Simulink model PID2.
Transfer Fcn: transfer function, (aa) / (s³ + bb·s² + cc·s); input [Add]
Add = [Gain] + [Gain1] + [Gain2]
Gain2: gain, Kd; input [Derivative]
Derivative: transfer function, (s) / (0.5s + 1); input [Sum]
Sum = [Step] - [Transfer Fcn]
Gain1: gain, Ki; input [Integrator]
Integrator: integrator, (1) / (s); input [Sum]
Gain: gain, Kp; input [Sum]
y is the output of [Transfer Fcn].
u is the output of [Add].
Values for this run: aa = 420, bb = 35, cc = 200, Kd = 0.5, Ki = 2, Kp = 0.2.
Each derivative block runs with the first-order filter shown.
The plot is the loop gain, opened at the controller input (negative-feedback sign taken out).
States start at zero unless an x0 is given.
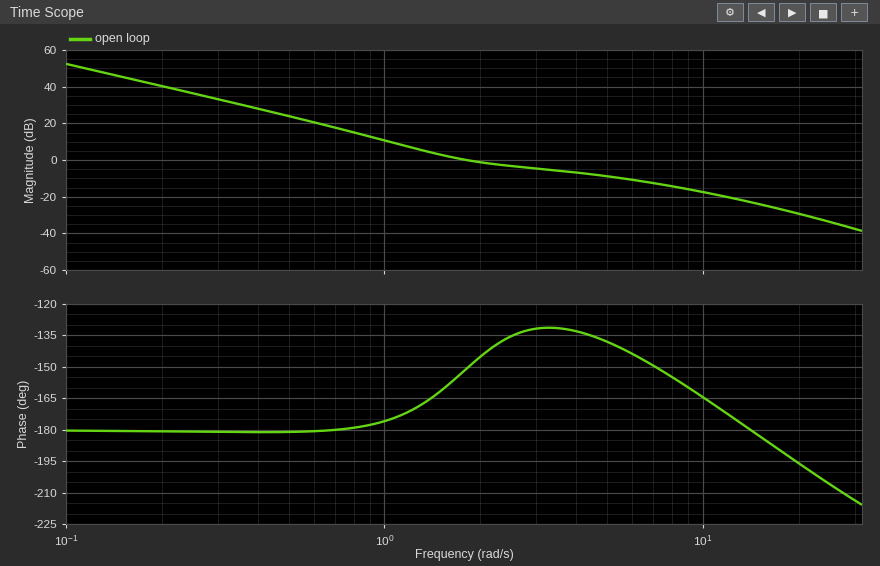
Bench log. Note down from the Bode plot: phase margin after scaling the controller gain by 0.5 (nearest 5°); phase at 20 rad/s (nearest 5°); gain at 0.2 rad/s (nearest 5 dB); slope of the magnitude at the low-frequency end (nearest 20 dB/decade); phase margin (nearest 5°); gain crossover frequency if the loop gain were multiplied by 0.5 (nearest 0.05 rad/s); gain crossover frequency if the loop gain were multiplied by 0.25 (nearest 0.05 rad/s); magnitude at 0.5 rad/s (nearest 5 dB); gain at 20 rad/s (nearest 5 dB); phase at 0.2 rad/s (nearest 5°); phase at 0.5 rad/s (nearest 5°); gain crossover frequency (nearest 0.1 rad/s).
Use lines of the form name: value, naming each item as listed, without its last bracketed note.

phase margin after scaling the controller gain by 0.5: 10°
phase at 20 rad/s: -195°
gain at 0.2 rad/s: 40 dB
slope of the magnitude at the low-frequency end: -40 dB/decade
phase margin: 30°
gain crossover frequency if the loop gain were multiplied by 0.5: 1.25 rad/s
gain crossover frequency if the loop gain were multiplied by 0.25: 0.95 rad/s
magnitude at 0.5 rad/s: 25 dB
gain at 20 rad/s: -30 dB
phase at 0.2 rad/s: -180°
phase at 0.5 rad/s: -180°
gain crossover frequency: 1.8 rad/s
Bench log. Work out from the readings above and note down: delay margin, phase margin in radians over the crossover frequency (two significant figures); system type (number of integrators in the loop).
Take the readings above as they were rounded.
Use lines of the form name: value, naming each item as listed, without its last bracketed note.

delay margin, phase margin in radians over the crossover frequency: 0.29 s
system type: 2
